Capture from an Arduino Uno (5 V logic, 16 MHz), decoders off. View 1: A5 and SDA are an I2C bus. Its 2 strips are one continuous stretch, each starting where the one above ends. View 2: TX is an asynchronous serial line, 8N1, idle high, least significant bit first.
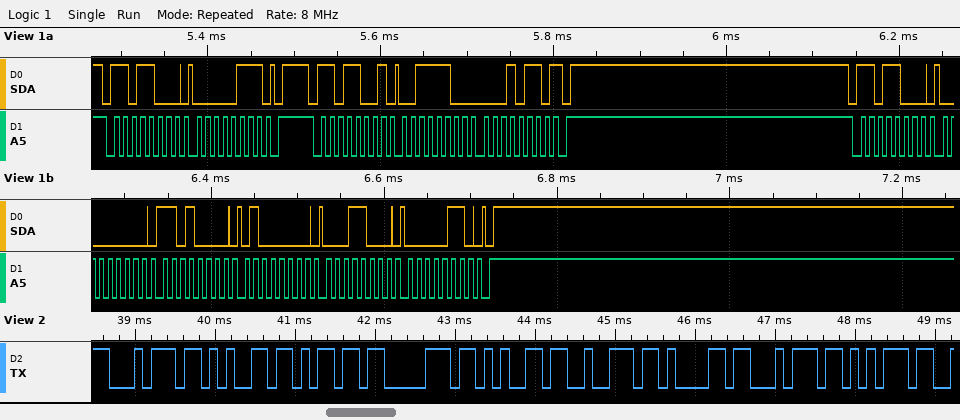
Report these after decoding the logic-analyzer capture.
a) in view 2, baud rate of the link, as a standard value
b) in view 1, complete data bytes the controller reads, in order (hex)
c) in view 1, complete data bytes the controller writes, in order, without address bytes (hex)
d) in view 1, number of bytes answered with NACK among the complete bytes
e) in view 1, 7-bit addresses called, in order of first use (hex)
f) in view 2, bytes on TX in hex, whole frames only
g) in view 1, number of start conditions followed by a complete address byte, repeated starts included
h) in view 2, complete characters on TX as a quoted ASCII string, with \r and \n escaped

9600 baud
3C 16
07 00 D0 40 18 06
1
0x6C
0x74 0x65 0x6D 0x70 0x65 0x72 0x61 0x74 0x75
3
"temperatu"
